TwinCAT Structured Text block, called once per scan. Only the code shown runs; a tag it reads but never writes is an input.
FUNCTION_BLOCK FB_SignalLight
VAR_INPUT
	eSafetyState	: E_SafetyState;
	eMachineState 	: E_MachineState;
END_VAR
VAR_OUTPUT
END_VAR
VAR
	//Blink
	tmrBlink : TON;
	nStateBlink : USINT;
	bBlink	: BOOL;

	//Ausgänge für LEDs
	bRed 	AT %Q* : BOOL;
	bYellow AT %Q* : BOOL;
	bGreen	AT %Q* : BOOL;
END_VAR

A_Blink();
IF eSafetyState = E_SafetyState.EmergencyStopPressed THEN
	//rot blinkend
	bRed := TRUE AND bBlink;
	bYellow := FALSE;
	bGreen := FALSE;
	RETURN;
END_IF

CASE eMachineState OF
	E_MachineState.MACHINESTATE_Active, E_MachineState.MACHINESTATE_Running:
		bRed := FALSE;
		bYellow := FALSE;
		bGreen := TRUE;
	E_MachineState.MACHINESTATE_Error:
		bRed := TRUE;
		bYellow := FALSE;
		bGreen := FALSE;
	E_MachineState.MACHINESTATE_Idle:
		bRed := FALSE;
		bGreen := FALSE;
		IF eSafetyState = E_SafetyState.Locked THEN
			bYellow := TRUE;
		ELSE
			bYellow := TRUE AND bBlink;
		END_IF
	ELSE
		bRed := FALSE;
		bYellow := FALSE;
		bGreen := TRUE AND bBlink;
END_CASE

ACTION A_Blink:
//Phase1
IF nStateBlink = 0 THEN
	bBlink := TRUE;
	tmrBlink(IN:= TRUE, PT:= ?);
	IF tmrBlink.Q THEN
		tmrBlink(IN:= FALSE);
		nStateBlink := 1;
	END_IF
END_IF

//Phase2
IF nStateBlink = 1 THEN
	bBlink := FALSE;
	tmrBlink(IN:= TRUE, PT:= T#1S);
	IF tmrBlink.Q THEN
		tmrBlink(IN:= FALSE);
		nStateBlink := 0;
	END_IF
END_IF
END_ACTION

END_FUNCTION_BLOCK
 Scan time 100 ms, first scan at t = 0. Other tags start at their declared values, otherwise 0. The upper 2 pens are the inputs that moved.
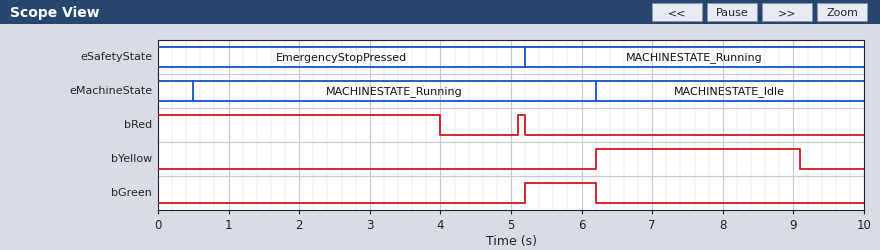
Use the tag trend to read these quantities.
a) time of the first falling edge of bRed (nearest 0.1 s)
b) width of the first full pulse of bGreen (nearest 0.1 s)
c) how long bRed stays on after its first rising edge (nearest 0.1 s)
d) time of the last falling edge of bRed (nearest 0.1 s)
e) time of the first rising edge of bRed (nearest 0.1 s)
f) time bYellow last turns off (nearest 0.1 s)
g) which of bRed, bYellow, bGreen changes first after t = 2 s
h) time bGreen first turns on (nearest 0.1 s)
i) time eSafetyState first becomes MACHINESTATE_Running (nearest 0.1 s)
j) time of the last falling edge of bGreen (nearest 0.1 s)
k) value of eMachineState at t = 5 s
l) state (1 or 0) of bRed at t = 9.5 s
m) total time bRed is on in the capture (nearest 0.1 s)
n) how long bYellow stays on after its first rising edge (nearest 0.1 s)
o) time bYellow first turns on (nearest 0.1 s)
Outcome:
4.0 s
1.0 s
0.1 s
5.2 s
5.1 s
9.1 s
bRed
5.2 s
5.2 s
6.2 s
MACHINESTATE_Running
0
4.1 s
2.9 s
6.2 s
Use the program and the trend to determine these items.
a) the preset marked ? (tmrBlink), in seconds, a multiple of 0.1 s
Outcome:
4.0 s
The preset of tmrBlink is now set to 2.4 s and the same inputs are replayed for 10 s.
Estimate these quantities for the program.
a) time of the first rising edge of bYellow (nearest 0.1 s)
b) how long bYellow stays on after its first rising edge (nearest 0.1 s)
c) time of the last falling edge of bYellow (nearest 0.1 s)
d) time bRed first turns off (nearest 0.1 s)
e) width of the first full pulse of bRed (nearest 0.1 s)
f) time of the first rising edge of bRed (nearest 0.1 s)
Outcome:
7.0 s
2.4 s
9.4 s
2.4 s
1.7 s
3.5 s
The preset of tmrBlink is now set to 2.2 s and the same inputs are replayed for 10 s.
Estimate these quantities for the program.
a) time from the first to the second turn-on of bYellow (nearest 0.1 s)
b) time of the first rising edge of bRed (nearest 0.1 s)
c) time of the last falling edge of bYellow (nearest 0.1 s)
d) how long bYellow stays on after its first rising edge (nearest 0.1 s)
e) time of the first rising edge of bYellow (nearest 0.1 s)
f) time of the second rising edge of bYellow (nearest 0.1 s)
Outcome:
3.3 s
3.3 s
8.8 s
2.2 s
6.6 s
9.9 s
